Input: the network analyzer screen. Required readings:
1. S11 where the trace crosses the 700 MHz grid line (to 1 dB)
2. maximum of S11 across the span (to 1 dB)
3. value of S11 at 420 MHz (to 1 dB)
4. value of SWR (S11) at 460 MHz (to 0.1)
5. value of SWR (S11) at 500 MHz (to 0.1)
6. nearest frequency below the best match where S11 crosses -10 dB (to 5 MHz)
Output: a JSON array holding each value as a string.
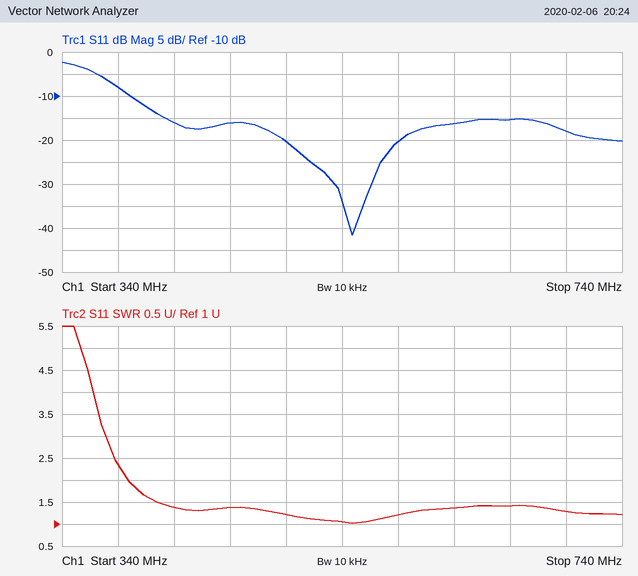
["-18 dB", "-2 dB", "-16 dB", "1.4", "1.2", "390 MHz"]
